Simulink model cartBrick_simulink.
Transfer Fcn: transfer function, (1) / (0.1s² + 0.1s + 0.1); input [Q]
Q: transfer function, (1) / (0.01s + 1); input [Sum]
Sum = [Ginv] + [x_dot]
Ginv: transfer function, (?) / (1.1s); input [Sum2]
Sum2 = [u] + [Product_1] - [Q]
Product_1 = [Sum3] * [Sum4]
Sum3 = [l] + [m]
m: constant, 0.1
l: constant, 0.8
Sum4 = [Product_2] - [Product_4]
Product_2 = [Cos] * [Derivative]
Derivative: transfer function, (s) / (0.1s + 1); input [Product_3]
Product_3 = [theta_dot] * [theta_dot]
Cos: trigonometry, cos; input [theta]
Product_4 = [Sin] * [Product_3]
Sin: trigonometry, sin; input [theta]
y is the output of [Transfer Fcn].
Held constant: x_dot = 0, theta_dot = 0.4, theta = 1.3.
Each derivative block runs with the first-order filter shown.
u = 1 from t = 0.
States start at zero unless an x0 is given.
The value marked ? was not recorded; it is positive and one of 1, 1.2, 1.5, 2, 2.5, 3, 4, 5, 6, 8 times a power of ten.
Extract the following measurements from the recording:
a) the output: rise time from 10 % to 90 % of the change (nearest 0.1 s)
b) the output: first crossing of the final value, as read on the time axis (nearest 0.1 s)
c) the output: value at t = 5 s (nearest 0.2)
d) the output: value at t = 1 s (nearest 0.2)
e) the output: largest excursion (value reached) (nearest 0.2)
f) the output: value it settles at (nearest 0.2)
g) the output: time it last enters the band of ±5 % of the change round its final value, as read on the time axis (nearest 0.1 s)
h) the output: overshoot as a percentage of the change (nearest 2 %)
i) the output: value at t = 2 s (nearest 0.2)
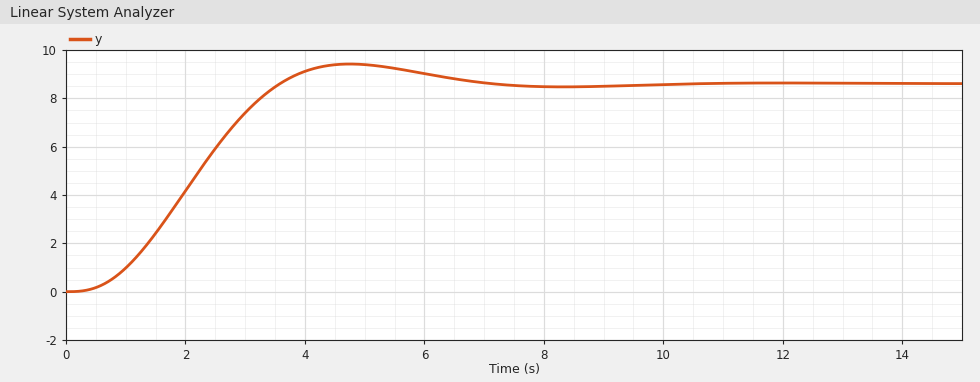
2.2 s
3.6 s
9.4
1.0
9.4
8.6
6.0 s
10 %
4.2
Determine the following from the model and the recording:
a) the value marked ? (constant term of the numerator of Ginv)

1.2
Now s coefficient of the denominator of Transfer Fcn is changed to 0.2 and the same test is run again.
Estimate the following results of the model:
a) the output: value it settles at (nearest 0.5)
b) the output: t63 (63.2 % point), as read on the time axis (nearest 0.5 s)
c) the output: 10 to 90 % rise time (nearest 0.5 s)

8.5
3.0 s
4.0 s
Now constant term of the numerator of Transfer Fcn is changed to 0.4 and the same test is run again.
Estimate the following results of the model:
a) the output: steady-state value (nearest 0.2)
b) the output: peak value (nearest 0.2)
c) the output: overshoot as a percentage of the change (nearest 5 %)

3.4
3.8
10 %
